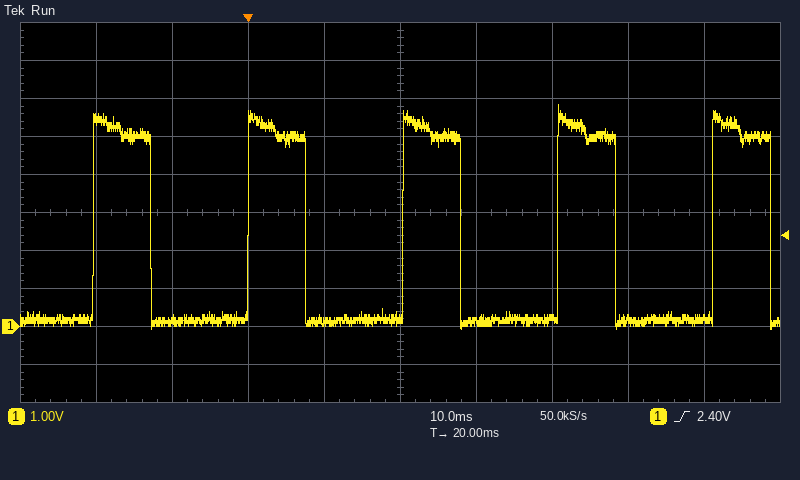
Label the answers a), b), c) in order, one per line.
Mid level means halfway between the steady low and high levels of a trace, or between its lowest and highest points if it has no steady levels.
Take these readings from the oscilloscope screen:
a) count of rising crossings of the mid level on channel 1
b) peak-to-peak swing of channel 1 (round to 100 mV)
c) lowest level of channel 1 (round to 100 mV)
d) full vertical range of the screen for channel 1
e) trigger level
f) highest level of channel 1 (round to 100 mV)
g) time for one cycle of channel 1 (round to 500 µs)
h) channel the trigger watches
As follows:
a) 5
b) 5.9 V
c) -100 mV
d) 10 V
e) 2.40 V
f) 5.8 V
g) 20.5 ms
h) channel 1
